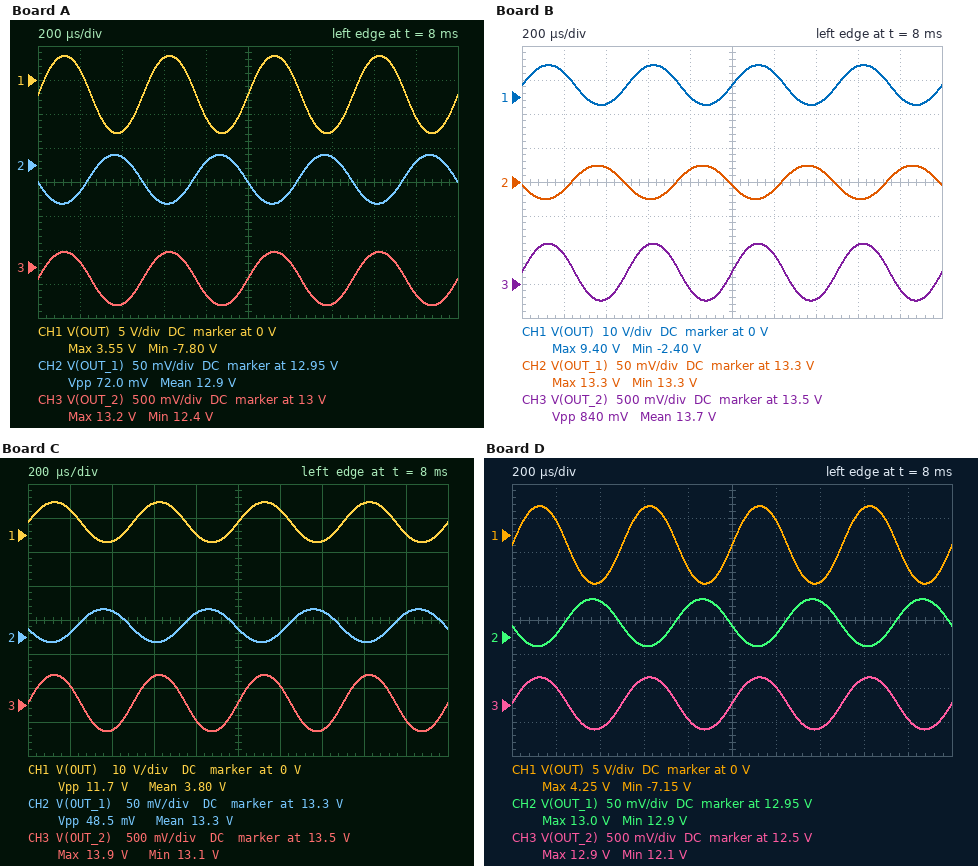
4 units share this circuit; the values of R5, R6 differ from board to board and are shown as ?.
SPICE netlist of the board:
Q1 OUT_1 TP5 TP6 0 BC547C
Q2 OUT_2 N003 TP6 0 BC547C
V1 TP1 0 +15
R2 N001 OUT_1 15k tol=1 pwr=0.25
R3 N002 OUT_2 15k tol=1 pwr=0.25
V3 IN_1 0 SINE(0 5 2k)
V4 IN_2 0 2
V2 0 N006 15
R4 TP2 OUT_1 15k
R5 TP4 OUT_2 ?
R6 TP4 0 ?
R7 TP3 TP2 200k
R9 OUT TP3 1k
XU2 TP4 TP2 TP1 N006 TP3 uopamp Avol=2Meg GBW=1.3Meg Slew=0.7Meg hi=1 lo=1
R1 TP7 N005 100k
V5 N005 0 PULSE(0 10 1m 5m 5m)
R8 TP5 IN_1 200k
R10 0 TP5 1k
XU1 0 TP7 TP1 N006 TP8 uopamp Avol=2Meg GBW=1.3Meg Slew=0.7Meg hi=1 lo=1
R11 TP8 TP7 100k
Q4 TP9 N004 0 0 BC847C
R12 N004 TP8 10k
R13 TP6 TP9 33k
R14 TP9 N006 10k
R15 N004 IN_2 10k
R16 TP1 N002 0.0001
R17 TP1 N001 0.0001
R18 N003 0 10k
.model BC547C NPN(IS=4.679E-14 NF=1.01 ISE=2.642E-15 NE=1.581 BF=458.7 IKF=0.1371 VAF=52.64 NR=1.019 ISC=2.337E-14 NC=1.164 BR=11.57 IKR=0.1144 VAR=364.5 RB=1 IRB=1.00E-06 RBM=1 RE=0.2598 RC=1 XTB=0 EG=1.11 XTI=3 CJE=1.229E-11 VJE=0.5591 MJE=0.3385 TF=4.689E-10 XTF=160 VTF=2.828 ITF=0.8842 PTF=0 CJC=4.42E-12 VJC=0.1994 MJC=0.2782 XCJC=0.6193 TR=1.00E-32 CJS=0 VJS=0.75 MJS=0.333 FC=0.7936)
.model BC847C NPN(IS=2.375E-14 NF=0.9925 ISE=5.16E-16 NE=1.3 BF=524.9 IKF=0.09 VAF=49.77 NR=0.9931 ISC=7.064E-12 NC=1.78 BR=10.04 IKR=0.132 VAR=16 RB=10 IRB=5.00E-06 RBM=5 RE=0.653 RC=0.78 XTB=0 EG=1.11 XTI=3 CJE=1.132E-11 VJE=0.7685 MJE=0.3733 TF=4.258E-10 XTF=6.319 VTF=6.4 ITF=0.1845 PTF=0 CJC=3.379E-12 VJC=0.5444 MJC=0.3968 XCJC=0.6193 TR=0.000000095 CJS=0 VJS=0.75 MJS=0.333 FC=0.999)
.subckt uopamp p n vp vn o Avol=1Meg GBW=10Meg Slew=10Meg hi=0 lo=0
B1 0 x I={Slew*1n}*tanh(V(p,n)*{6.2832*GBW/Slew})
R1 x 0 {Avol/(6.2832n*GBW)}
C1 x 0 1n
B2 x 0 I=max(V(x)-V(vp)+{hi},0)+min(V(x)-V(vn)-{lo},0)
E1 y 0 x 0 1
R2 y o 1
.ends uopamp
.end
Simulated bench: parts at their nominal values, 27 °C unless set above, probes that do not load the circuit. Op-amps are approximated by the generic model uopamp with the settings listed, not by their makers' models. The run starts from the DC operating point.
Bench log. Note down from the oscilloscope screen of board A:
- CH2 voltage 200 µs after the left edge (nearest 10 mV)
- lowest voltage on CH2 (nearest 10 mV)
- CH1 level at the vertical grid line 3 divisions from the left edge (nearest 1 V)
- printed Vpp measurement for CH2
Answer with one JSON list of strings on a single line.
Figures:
["12.91 V", "12.89 V", "3 V", "72.0 mV"]
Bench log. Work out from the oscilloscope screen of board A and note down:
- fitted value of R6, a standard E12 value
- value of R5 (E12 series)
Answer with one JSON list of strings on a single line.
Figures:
["150 kΩ", "12 kΩ"]
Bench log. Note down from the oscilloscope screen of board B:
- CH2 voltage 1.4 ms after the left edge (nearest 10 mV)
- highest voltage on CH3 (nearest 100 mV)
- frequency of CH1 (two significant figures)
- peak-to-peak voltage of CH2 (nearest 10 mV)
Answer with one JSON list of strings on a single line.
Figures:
["13.32 V", "14.1 V", "2.0 kHz", "50 mV"]
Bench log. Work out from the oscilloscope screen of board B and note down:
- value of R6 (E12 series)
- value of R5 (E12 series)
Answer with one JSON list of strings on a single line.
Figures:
["560 kΩ", "47 kΩ"]
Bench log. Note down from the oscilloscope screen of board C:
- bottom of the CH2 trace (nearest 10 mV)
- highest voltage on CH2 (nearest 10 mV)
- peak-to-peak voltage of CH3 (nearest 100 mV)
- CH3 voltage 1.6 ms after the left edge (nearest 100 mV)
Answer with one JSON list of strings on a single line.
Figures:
["13.29 V", "13.34 V", "800 mV", "13.9 V"]
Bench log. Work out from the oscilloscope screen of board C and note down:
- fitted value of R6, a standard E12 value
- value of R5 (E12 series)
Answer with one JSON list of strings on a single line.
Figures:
["390 kΩ", "27 kΩ"]
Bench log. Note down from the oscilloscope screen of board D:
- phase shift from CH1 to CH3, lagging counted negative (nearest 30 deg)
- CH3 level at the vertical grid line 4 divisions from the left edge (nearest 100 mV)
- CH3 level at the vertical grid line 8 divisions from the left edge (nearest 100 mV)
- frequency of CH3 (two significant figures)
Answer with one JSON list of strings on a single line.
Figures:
["0 deg", "12.3 V", "12.9 V", "2.0 kHz"]
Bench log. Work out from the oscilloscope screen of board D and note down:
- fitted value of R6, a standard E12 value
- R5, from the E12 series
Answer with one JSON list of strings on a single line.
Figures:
["120 kΩ", "5.6 kΩ"]
